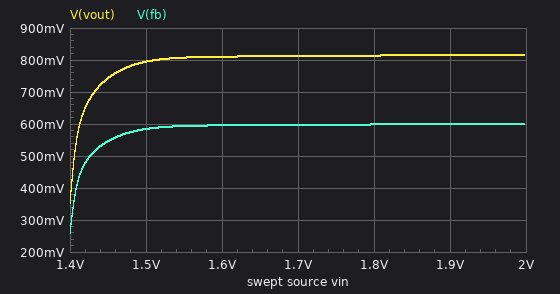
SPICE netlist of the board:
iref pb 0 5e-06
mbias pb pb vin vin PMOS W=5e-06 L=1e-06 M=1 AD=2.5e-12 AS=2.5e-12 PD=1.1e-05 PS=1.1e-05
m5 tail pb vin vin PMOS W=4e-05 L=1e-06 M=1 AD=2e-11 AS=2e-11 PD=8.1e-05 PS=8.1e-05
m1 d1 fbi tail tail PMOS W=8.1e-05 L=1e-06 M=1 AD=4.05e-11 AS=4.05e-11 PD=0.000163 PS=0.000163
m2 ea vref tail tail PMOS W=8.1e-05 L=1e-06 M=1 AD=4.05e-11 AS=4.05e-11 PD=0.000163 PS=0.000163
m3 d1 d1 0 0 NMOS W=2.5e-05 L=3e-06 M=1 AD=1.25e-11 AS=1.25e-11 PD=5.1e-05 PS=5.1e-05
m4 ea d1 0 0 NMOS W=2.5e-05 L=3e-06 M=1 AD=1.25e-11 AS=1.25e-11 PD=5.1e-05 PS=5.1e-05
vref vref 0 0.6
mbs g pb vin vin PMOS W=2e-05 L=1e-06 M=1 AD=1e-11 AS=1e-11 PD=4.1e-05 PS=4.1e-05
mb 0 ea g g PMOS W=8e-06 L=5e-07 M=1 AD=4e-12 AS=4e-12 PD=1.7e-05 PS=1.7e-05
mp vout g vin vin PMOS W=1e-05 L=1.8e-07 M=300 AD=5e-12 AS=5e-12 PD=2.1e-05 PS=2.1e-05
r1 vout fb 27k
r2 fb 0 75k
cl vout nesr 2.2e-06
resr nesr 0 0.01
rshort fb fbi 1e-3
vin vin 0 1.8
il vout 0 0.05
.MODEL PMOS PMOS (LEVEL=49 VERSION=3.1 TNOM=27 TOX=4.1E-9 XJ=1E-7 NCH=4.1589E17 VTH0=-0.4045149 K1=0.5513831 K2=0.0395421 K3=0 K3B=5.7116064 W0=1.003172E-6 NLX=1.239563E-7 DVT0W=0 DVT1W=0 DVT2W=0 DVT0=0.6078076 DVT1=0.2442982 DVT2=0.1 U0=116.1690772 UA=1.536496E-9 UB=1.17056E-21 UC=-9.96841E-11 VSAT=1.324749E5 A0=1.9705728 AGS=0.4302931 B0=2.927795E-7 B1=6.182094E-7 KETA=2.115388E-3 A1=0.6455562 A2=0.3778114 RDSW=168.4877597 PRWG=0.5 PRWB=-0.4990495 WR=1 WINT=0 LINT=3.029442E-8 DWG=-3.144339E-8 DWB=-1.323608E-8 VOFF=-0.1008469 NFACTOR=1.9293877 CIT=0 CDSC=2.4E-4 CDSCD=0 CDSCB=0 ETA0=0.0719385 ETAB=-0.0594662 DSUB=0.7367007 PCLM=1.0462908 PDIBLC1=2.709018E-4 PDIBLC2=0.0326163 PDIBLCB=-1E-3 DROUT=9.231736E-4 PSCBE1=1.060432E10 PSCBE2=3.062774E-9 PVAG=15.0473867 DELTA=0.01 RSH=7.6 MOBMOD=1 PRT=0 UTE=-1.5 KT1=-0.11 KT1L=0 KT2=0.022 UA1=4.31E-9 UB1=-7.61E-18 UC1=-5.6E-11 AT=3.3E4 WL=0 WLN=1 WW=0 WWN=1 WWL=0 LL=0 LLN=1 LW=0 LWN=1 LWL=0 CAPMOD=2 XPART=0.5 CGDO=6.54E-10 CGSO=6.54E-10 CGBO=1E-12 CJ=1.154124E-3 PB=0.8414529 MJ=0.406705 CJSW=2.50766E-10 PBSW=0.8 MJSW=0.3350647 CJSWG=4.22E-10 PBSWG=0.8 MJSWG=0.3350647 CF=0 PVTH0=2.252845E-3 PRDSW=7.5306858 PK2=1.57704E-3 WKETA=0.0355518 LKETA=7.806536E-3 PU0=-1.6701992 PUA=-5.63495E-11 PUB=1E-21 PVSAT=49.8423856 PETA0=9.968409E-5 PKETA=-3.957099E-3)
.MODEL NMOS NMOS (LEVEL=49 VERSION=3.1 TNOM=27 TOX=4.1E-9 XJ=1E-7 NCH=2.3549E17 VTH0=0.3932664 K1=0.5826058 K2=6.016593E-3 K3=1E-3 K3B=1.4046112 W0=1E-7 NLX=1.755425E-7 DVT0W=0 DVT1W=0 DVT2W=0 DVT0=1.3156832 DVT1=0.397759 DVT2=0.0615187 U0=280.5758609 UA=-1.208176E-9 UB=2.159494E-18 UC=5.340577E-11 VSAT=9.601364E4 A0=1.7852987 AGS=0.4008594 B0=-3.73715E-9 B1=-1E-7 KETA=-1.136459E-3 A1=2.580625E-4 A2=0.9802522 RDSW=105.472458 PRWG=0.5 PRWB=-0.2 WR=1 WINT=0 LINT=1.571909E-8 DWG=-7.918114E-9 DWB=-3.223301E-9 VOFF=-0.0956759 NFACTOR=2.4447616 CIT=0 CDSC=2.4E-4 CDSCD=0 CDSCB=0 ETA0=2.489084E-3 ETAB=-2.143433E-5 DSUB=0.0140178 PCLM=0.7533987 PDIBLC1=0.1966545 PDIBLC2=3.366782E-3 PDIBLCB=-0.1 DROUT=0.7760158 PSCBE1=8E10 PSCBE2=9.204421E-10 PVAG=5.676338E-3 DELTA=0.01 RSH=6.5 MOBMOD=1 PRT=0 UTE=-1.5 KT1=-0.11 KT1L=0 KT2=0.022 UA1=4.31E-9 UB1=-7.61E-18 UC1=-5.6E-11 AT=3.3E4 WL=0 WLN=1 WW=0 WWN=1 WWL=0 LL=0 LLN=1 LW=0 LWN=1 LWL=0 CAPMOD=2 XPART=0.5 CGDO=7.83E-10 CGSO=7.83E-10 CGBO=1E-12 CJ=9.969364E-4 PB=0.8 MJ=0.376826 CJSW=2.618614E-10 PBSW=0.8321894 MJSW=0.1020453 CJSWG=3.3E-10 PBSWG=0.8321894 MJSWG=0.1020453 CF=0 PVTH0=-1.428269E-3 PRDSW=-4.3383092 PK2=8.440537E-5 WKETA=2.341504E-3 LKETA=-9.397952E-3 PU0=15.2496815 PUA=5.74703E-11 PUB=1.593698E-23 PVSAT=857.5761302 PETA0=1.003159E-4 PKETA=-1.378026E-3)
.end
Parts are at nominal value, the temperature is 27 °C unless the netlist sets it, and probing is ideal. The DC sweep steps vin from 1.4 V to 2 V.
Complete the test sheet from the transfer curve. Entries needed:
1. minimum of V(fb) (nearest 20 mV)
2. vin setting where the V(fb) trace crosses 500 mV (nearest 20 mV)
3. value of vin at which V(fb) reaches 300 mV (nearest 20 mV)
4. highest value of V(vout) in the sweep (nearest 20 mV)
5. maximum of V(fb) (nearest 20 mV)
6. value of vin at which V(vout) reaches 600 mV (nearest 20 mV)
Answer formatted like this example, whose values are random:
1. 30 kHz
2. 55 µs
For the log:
1. 260 mV
2. 1.42 V
3. 1.40 V
4. 820 mV
5. 600 mV
6. 1.42 V
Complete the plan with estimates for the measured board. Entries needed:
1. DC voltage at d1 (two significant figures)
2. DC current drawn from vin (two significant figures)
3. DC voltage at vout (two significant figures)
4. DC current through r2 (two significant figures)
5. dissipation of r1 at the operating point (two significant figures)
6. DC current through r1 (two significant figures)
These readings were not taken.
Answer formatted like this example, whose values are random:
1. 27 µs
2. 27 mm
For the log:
1. 560 mV
2. 50 mA
3. 810 mV
4. 8.0 µA
5. 1.7 µW
6. 8.0 µA
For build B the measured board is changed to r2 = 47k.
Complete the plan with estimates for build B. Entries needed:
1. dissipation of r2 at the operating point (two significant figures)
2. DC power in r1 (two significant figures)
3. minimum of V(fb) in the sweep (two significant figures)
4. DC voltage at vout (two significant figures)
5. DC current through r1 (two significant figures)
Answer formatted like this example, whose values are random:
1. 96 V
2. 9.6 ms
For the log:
1. 7.6 µW
2. 4.4 µW
3. 220 mV
4. 940 mV
5. 13 µA
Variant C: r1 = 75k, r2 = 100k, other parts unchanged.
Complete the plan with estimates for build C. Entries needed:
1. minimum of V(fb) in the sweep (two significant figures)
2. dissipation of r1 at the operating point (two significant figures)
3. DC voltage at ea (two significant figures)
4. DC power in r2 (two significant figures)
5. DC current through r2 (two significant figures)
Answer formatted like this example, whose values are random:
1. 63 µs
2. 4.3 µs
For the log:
1. 200 mV
2. 2.7 µW
3. 390 mV
4. 3.6 µW
5. 6.0 µA
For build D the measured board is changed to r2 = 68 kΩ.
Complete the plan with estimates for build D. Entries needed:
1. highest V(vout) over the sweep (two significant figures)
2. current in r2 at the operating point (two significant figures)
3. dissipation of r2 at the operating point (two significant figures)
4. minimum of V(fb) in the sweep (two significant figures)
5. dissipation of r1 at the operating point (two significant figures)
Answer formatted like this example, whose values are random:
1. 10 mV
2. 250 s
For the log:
1. 840 mV
2. 8.8 µA
3. 5.3 µW
4. 250 mV
5. 2.1 µW
